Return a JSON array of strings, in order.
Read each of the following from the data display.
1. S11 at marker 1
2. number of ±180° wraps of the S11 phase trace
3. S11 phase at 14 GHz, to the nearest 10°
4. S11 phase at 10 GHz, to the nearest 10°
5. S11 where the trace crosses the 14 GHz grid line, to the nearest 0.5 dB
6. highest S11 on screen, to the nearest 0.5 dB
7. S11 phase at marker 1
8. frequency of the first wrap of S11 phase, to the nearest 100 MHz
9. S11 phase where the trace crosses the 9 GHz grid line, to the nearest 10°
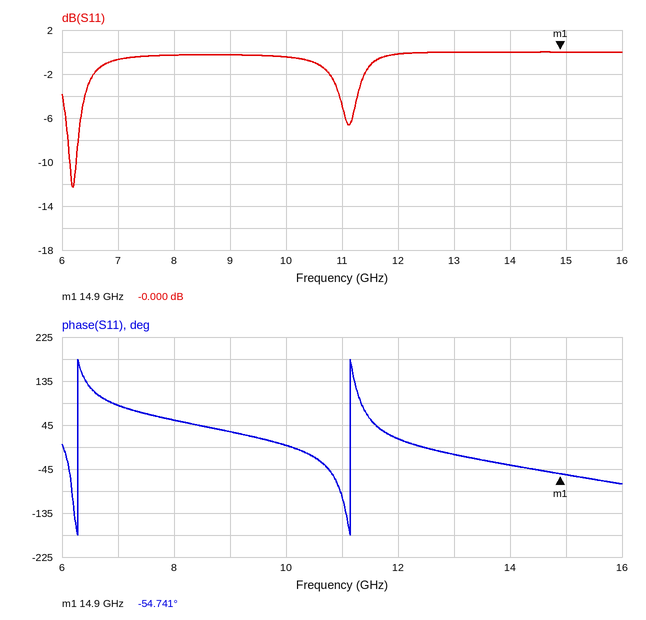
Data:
["-0.000 dB", "2", "-40°", "0°", "0.0 dB", "0.0 dB", "-54.741°", "6.3 GHz", "30°"]
